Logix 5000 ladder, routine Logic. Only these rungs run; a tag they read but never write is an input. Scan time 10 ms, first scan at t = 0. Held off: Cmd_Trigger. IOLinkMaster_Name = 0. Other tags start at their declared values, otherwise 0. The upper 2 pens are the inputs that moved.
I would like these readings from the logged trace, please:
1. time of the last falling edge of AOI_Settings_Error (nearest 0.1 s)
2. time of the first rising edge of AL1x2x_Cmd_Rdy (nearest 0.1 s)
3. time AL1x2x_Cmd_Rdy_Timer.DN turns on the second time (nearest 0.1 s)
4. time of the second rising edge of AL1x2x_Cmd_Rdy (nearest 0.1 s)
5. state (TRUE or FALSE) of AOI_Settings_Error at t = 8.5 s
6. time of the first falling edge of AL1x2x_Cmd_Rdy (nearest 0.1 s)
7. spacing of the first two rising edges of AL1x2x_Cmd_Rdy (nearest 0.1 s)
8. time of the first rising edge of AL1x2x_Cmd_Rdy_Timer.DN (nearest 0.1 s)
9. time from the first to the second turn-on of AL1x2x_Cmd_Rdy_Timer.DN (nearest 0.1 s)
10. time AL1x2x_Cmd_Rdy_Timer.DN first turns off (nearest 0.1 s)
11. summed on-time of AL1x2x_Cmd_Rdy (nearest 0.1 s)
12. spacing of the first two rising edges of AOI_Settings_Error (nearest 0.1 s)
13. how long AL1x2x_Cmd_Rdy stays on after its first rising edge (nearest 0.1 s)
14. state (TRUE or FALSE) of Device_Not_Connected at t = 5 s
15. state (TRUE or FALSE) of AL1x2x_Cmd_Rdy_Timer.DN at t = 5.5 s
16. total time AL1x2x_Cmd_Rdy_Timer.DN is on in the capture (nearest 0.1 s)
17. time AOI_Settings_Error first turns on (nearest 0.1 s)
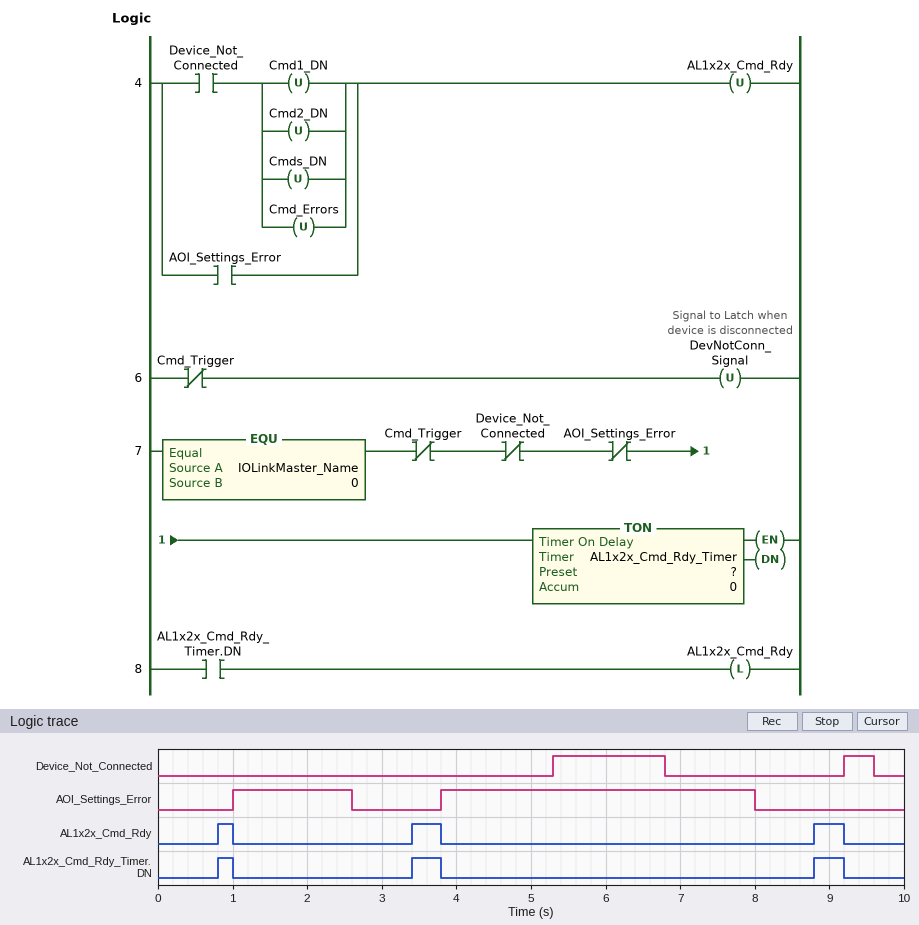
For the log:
8.0 s
0.8 s
3.4 s
3.4 s
FALSE
1.0 s
2.6 s
0.8 s
2.6 s
1.0 s
1.0 s
2.8 s
0.2 s
FALSE
FALSE
1.0 s
1.0 s
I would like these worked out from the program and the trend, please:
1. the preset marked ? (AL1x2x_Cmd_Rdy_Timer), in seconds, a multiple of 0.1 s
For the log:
0.8 s
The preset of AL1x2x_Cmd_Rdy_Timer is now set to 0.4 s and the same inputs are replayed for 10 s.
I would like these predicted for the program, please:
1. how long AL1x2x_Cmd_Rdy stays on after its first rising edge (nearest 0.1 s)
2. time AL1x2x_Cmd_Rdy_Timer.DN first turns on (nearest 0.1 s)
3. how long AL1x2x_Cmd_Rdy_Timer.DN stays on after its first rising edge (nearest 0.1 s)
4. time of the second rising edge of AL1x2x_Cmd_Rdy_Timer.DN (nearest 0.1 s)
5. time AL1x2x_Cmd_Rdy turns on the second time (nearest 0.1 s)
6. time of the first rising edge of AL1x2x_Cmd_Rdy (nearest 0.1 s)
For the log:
0.6 s
0.4 s
0.6 s
3.0 s
3.0 s
0.4 s
